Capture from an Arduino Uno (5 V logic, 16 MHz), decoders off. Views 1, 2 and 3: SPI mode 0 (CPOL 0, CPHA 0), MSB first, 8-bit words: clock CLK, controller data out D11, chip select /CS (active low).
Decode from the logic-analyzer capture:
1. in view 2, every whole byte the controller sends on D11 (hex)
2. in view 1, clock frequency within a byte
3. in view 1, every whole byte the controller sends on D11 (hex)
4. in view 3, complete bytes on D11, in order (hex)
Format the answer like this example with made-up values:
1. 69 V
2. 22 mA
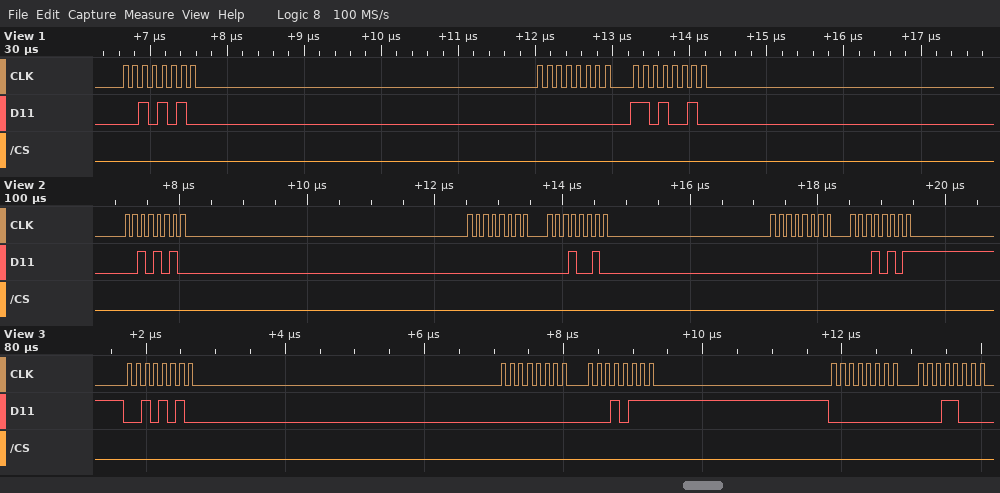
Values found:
1. 2A 00 12 00 15
2. 8 MHz
3. 0x2A 0x00 0xD2
4. 2A 00 17 00 18
